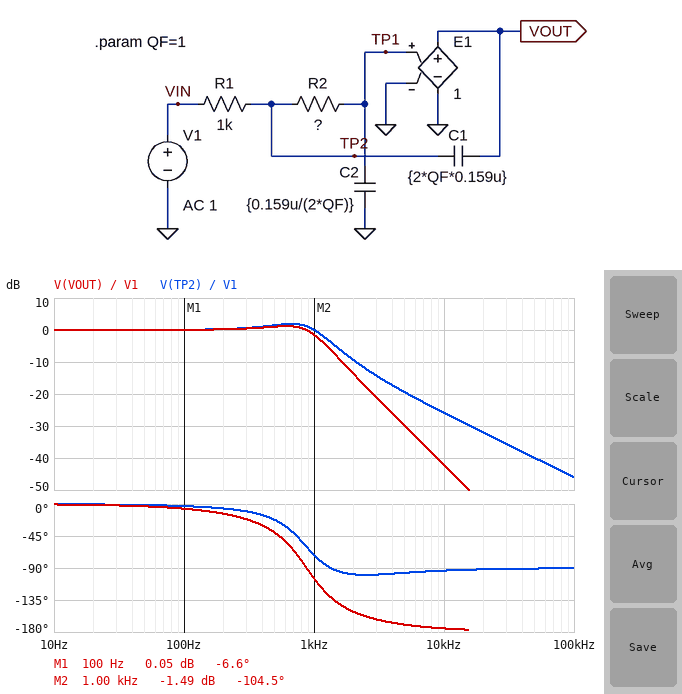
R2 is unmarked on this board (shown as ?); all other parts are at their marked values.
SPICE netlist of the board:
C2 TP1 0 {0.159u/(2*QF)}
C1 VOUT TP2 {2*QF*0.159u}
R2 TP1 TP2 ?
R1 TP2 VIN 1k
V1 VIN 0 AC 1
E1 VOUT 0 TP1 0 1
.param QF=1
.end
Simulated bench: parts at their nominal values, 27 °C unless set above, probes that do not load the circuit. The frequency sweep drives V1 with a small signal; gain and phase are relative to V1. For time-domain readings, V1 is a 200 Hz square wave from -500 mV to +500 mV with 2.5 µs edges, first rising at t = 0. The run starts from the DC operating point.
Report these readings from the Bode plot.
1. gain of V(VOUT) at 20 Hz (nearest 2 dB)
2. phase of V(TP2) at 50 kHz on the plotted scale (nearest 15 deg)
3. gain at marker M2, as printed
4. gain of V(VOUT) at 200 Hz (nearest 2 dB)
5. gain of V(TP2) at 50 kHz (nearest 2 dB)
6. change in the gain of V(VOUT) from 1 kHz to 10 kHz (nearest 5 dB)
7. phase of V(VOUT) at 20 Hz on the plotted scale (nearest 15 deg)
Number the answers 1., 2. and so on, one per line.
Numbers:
1. 0 dB
2. -90 deg
3. -1.49 dB
4. 0 dB
5. -40 dB
6. -40 dB
7. 0 deg
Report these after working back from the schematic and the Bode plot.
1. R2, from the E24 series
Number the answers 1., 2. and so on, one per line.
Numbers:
1. 1.3 kΩ
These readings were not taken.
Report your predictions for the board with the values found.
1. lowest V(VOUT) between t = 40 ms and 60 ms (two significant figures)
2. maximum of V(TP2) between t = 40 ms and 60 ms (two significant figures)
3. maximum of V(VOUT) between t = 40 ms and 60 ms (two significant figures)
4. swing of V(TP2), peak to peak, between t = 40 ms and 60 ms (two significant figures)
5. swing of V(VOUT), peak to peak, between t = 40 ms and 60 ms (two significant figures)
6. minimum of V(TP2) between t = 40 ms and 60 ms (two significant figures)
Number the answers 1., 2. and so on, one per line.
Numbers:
1. -660 mV
2. 700 mV
3. 660 mV
4. 1.4 V
5. 1.3 V
6. -700 mV
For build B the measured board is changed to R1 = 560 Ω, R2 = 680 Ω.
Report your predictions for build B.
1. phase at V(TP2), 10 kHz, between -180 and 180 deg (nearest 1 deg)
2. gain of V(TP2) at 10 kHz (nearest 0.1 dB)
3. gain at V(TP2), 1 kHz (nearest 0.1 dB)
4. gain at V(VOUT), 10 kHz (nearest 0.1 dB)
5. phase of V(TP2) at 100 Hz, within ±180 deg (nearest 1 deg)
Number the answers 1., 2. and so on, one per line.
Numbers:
1. -97 deg
2. -20.5 dB
3. 1.6 dB
4. -31.5 dB
5. -2 deg
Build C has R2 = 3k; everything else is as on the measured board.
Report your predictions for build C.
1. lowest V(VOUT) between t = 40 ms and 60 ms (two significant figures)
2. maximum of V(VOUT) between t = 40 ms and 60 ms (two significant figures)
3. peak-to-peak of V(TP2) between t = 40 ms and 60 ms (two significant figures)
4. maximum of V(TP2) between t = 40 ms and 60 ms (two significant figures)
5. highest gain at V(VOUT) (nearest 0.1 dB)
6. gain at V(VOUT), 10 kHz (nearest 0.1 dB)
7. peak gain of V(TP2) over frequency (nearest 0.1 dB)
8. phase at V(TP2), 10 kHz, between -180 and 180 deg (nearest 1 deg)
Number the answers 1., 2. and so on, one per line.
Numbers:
1. -610 mV
2. 610 mV
3. 1.4 V
4. 680 mV
5. 0.5 dB
6. -49.5 dB
7. 1.8 dB
8. -90 deg
